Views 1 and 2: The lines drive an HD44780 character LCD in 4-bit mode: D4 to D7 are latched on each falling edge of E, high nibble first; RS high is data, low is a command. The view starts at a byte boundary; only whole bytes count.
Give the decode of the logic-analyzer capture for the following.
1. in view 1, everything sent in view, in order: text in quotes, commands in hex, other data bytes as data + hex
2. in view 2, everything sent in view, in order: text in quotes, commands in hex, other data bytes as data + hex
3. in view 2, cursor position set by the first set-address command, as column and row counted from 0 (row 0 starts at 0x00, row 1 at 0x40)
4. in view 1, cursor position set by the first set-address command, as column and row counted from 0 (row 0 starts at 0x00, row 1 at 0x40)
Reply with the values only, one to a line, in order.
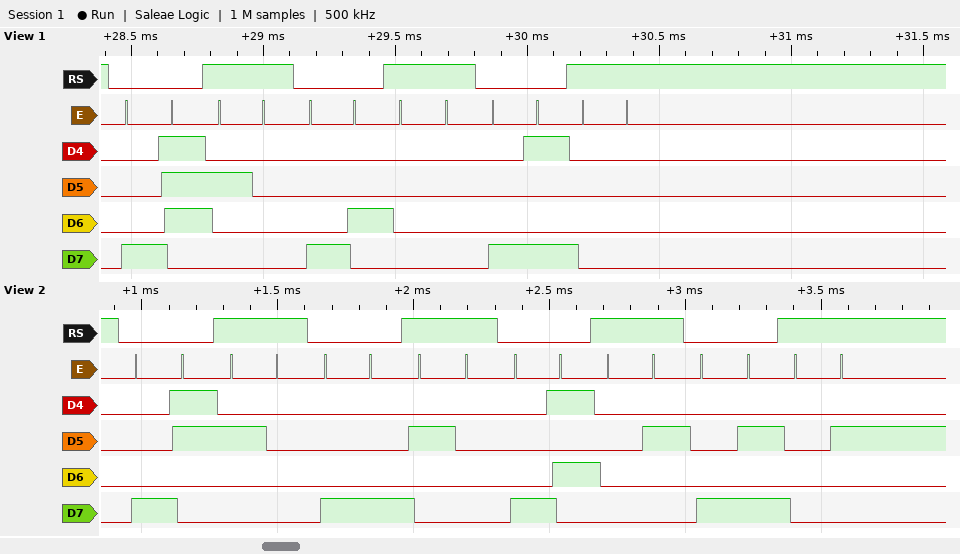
0x87 " " 0x84 data 00 0x89 data 00
0x83 " " 0x88 " " 0x85 data 02 0x8A data 02
column 3, row 0
column 7, row 0
